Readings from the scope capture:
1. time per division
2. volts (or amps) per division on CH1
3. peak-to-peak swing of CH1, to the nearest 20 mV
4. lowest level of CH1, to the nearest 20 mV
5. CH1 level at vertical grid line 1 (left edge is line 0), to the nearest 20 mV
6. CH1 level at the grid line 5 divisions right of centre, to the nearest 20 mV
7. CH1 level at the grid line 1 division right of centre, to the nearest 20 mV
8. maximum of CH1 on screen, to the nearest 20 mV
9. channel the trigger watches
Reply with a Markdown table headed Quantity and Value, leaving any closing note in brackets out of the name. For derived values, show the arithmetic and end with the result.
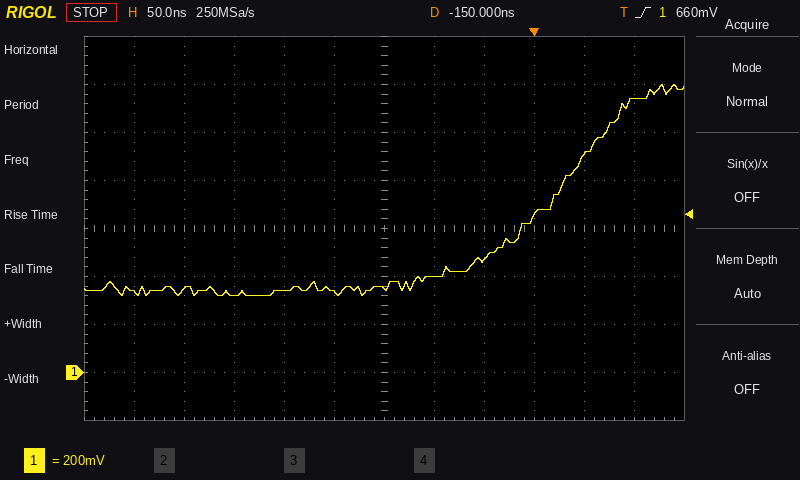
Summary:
| Quantity | Value |
|---|---|
| time per division | 50 ns |
| volts (or amps) per division on CH1 | 200 mV |
| peak-to-peak swing of CH1, to the nearest 20 mV | 1.20 V − (320 mV) = 880 mV |
| lowest level of CH1, to the nearest 20 mV | 320 mV |
| CH1 level at vertical grid line 1 (left edge is line 0), to the nearest 20 mV | 340 mV |
| CH1 level at the grid line 5 divisions right of centre, to the nearest 20 mV | 1.14 V |
| CH1 level at the grid line 1 division right of centre, to the nearest 20 mV | 400 mV |
| maximum of CH1 on screen, to the nearest 20 mV | 1.20 V |
| channel the trigger watches | CH1 |
